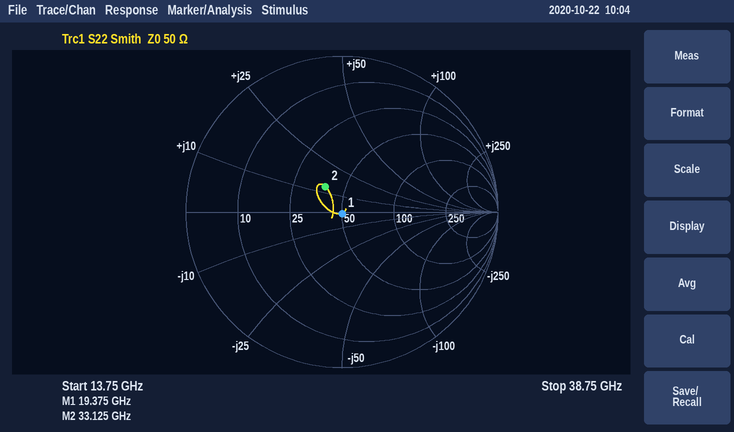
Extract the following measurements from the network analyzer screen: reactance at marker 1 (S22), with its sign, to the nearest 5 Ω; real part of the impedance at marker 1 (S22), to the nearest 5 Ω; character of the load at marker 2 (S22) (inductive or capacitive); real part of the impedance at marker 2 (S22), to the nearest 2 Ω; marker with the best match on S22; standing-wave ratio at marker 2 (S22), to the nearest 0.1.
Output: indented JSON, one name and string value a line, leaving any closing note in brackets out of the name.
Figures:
{
  "reactance at marker 1 (S22), with its sign, to the nearest 5 Ω": "0 Ω",
  "real part of the impedance at marker 1 (S22), to the nearest 5 Ω": "50 Ω",
  "character of the load at marker 2 (S22)": "inductive",
  "real part of the impedance at marker 2 (S22), to the nearest 2 Ω": "38 Ω",
  "marker with the best match on S22": "marker 1",
  "standing-wave ratio at marker 2 (S22), to the nearest 0.1": "1.5"
}
